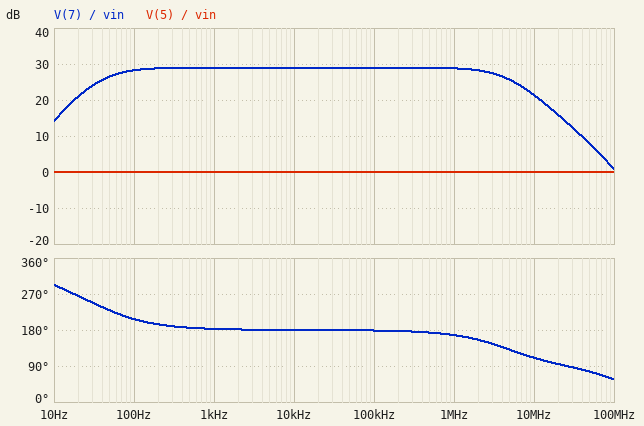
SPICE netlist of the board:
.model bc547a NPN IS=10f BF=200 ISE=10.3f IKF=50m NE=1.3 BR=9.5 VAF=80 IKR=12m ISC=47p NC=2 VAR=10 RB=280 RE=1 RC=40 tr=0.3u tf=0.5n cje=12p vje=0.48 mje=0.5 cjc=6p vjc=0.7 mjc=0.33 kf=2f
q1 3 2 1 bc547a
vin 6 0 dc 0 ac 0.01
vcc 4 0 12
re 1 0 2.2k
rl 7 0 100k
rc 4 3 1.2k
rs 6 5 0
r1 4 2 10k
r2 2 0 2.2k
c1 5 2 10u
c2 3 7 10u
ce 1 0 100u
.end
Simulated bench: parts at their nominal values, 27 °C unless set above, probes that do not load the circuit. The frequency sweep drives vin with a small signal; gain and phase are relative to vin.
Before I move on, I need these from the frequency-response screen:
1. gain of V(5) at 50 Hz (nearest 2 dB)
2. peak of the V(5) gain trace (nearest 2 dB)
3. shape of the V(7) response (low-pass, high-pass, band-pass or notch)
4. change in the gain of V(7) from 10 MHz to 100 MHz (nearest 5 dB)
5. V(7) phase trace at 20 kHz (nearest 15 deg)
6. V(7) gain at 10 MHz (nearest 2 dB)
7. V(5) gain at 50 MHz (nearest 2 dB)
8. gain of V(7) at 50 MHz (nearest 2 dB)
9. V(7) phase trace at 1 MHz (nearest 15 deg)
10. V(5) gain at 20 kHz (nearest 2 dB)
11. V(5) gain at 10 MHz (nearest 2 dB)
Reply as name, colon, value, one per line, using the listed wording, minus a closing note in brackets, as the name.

gain of V(5) at 50 Hz: 0 dB
peak of the V(5) gain trace: 0 dB
shape of the V(7) response: band-pass
change in the gain of V(7) from 10 MHz to 100 MHz: -20 dB
V(7) phase trace at 20 kHz: 180 deg
V(7) gain at 10 MHz: 22 dB
V(5) gain at 50 MHz: 0 dB
gain of V(7) at 50 MHz: 8 dB
V(7) phase trace at 1 MHz: 165 deg
V(5) gain at 20 kHz: 0 dB
V(5) gain at 10 MHz: 0 dB
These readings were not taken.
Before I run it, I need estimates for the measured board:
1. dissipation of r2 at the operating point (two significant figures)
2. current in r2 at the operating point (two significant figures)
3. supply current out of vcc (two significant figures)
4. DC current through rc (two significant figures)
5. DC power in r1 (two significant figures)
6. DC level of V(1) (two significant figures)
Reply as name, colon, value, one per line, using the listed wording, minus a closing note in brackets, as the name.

dissipation of r2 at the operating point: 2.1 mW
current in r2 at the operating point: 980 µA
supply current out of vcc: 1.7 mA
DC current through rc: 680 µA
DC power in r1: 9.7 mW
DC level of V(1): 1.5 V
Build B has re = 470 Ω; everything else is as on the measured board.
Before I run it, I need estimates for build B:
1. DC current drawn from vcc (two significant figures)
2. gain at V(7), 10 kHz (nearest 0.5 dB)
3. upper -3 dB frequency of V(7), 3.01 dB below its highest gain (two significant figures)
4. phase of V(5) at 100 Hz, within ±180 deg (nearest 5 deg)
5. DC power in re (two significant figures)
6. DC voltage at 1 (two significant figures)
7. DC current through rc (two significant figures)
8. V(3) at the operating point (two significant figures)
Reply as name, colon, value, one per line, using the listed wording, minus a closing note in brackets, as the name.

DC current drawn from vcc: 4.0 mA
gain at V(7), 10 kHz: 39.5 dB
upper -3 dB frequency of V(7), 3.01 dB below its highest gain: 1.6 MHz
phase of V(5) at 100 Hz, within ±180 deg: 0 deg
DC power in re: 4.3 mW
DC voltage at 1: 1.4 V
DC current through rc: 3.0 mA
V(3) at the operating point: 8.4 V
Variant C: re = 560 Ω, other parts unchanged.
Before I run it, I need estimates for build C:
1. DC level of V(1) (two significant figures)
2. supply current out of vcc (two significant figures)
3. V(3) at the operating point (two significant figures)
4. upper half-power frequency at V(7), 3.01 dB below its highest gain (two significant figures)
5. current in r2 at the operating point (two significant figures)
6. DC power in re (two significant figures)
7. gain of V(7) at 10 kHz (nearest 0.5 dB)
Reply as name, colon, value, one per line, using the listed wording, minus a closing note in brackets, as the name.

DC level of V(1): 1.4 V
supply current out of vcc: 3.5 mA
V(3) at the operating point: 8.9 V
upper half-power frequency at V(7), 3.01 dB below its highest gain: 1.8 MHz
current in r2 at the operating point: 970 µA
DC power in re: 3.7 mW
gain of V(7) at 10 kHz: 38.5 dB
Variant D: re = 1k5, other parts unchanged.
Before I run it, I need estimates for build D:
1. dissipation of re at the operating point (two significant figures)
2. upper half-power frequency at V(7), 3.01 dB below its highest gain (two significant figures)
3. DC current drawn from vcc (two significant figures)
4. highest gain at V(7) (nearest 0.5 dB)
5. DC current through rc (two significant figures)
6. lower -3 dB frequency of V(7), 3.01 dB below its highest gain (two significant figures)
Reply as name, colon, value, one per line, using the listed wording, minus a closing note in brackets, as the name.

dissipation of re at the operating point: 1.5 mW
upper half-power frequency at V(7), 3.01 dB below its highest gain: 3.6 MHz
DC current drawn from vcc: 2.0 mA
highest gain at V(7): 32.0 dB
DC current through rc: 990 µA
lower -3 dB frequency of V(7), 3.01 dB below its highest gain: 60 Hz
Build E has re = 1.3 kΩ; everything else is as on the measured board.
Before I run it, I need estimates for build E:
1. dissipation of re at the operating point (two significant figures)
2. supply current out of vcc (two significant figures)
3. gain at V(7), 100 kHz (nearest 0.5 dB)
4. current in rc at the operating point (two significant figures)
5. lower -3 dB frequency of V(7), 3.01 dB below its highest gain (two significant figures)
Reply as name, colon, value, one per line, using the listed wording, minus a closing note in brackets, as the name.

dissipation of re at the operating point: 1.7 mW
supply current out of vcc: 2.1 mA
gain at V(7), 100 kHz: 33.0 dB
current in rc at the operating point: 1.1 mA
lower -3 dB frequency of V(7), 3.01 dB below its highest gain: 67 Hz
